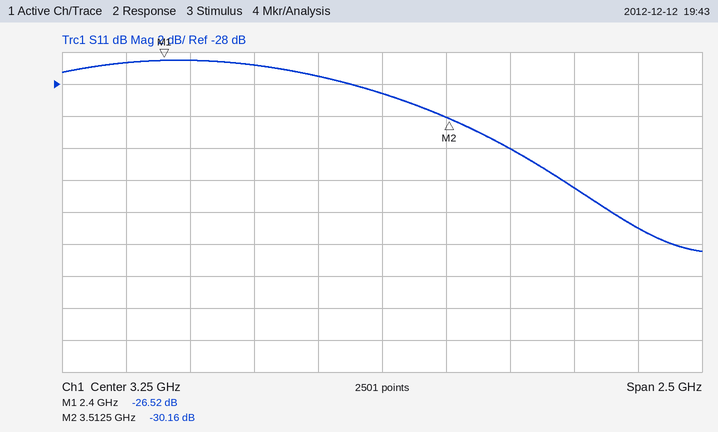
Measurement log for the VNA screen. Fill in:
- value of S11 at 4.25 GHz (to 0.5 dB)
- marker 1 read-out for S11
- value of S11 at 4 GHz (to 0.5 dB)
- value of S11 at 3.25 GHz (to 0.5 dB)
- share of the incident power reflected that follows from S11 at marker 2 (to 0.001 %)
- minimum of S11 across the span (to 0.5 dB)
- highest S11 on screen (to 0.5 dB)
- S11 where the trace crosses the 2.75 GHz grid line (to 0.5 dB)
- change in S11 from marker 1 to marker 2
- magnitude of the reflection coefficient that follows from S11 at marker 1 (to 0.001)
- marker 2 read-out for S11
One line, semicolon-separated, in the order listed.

-37.0 dB; -26.52 dB; -34.5 dB; -28.5 dB; 0.096 %; -38.5 dB; -26.5 dB; -27.0 dB; -3.64 dB; 0.047; -30.16 dB
